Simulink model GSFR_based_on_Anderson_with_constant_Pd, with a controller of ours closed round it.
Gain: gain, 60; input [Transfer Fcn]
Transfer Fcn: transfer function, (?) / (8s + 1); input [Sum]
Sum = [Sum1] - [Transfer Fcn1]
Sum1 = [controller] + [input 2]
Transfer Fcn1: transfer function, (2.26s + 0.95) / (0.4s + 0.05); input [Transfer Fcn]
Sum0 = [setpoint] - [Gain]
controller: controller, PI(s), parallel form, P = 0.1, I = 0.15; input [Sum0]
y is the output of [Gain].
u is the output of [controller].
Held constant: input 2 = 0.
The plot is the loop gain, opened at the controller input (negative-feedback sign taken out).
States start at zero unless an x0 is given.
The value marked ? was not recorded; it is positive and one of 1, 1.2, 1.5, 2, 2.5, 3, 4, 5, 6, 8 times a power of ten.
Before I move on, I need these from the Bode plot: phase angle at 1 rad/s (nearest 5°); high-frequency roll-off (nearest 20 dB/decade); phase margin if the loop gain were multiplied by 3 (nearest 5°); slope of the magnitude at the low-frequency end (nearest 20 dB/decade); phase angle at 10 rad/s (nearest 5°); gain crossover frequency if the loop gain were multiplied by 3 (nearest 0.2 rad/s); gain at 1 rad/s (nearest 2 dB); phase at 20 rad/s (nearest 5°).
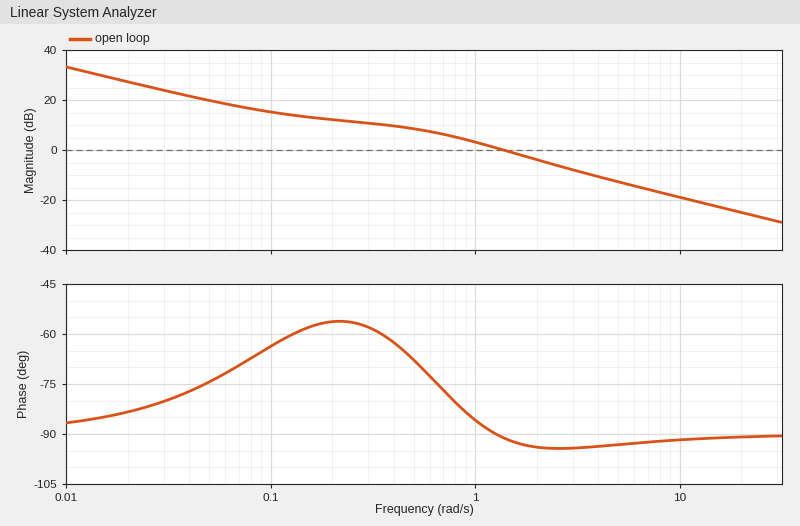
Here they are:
-85°
-20 dB/decade
85°
-20 dB/decade
-90°
3.6 rad/s
4 dB
-90°
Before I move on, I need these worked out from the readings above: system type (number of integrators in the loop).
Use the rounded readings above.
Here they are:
1
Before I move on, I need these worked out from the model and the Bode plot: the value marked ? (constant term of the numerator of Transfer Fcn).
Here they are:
1.5
